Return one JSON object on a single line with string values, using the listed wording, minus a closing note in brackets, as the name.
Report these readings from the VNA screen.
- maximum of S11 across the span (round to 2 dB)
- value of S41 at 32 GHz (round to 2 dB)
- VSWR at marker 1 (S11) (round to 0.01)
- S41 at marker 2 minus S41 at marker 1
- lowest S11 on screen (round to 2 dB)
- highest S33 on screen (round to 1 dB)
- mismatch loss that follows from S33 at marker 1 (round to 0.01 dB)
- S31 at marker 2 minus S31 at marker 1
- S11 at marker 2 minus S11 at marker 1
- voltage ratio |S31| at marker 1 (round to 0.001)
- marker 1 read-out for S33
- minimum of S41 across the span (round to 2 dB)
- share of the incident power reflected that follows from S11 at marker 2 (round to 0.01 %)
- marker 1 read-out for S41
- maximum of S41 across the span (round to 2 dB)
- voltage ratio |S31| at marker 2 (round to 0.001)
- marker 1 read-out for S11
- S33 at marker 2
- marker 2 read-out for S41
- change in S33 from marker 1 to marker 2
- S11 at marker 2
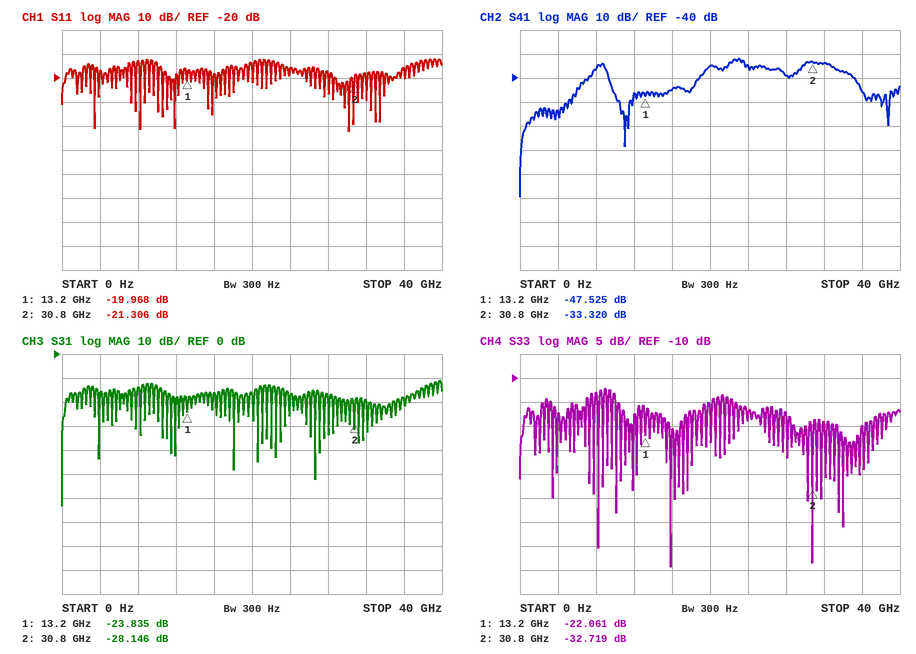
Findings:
{"maximum of S11 across the span": "-12 dB", "value of S41 at 32 GHz": "-34 dB", "VSWR at marker 1 (S11)": "1.22", "S41 at marker 2 minus S41 at marker 1": "14.205 dB", "lowest S11 on screen": "-42 dB", "highest S33 on screen": "-12 dB", "mismatch loss that follows from S33 at marker 1": "0.03 dB", "S31 at marker 2 minus S31 at marker 1": "-4.311 dB", "S11 at marker 2 minus S11 at marker 1": "-1.338 dB", "voltage ratio |S31| at marker 1": "0.064", "marker 1 read-out for S33": "-22.061 dB", "minimum of S41 across the span": "-90 dB", "share of the incident power reflected that follows from S11 at marker 2": "0.74 %", "marker 1 read-out for S41": "-47.525 dB", "maximum of S41 across the span": "-32 dB", "voltage ratio |S31| at marker 2": "0.039", "marker 1 read-out for S11": "-19.968 dB", "S33 at marker 2": "-32.719 dB", "marker 2 read-out for S41": "-33.320 dB", "change in S33 from marker 1 to marker 2": "-10.658 dB", "S11 at marker 2": "-21.306 dB"}
